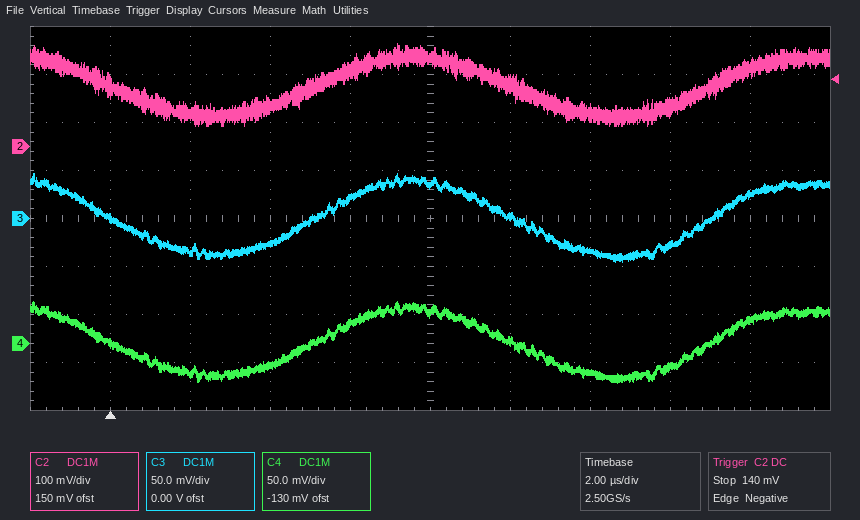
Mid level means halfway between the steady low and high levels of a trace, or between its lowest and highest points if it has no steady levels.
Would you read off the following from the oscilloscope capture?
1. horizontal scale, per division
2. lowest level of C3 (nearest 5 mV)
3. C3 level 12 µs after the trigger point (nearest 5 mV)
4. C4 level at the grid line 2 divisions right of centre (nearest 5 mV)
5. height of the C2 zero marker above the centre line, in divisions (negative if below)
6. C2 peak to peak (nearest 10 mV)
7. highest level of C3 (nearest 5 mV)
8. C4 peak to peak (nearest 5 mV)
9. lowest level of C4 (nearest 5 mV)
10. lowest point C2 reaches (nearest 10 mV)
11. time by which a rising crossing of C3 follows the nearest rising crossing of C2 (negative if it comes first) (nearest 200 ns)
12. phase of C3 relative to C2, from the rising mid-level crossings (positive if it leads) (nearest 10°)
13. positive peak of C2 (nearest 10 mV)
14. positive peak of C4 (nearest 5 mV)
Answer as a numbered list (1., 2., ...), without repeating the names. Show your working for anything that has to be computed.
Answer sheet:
1. 2 µs
2. -45 mV
3. -35 mV
4. -30 mV
5. +1.5 div
6. 210 mV − (40 mV) = 170 mV
7. 45 mV
8. 45 mV − (-40 mV) = 85 mV
9. -40 mV
10. 40 mV
11. 0.0 µs
12. 0°
13. 210 mV
14. 45 mV
